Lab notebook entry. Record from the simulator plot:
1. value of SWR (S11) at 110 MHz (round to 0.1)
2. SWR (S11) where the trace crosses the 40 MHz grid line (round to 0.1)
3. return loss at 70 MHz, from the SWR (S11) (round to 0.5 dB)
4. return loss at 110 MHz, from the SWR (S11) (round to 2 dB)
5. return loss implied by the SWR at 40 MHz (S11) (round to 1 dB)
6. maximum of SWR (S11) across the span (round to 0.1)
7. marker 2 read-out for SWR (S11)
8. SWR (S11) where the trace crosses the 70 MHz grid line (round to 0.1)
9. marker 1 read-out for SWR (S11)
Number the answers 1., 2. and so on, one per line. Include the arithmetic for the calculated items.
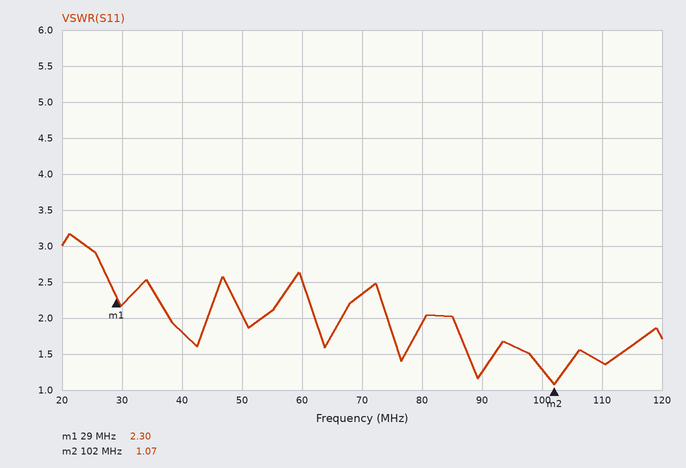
1. 1.4
2. 1.8
3. −20 log10((2.3 − 1)/(2.3 + 1)) ≈ 8.09 dB, so 8.0 dB to the nearest 0.5 dB
4. −20 log10((1.4 − 1)/(1.4 + 1)) ≈ 16 dB
5. −20 log10((1.8 − 1)/(1.8 + 1)) ≈ 11 dB
6. 3.2
7. 1.07
8. 2.3
9. 2.30
